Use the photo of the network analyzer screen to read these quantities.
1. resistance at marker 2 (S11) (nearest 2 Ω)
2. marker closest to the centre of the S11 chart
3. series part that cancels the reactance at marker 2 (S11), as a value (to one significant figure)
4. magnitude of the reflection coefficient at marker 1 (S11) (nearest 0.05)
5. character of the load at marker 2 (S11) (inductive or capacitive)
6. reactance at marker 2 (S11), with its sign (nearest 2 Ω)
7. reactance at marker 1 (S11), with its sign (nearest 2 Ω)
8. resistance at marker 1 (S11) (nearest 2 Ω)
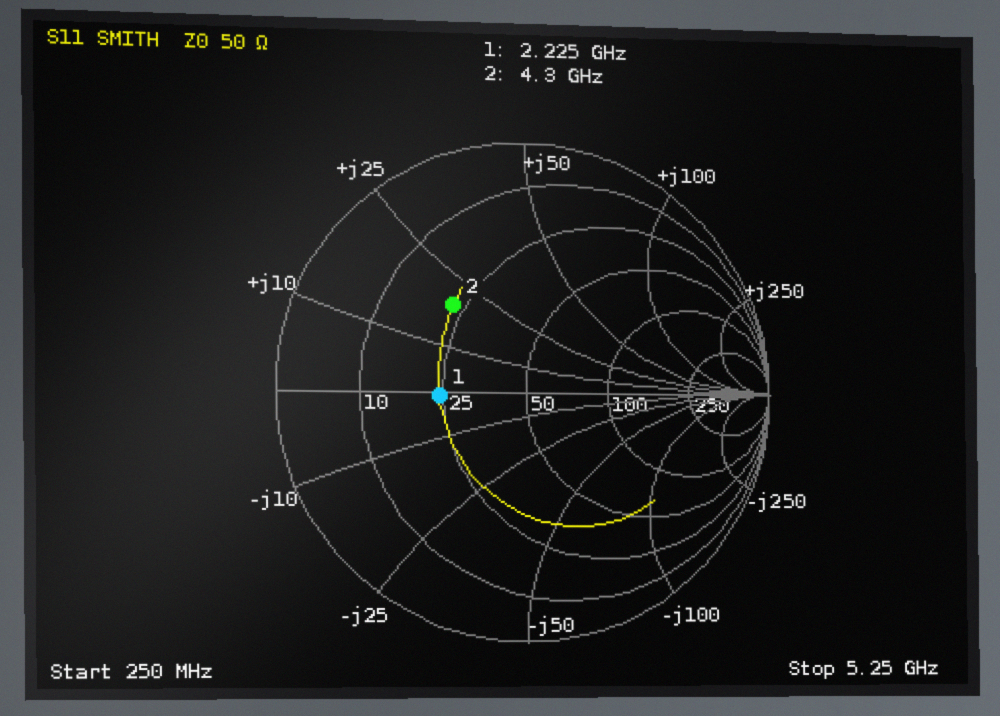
22 Ω
marker 1
2 pF
0.35
inductive
+20 Ω
0 Ω
24 Ω
